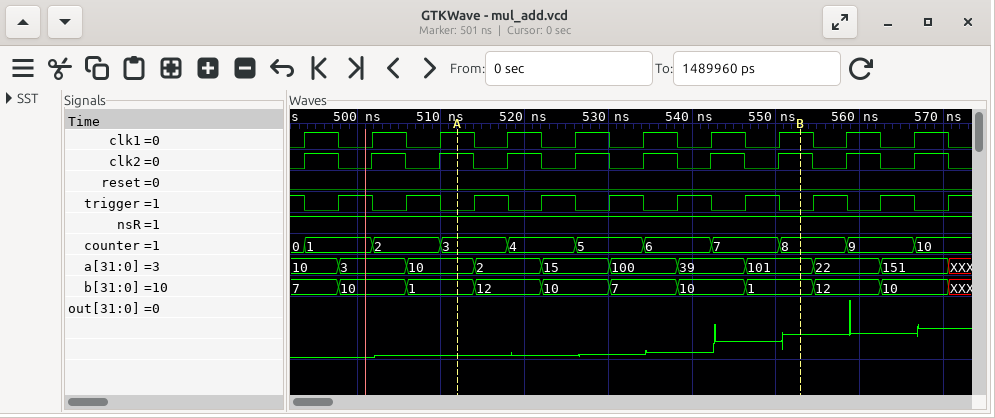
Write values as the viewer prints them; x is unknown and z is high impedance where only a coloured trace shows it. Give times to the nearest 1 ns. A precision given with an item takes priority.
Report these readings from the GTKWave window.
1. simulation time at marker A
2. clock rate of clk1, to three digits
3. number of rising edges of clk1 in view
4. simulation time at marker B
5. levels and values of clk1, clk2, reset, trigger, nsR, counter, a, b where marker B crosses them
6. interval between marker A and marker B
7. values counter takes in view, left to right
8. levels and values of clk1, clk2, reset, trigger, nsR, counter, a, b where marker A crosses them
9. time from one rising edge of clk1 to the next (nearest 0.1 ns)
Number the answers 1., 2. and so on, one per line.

1. 512 ns
2. 123 MHz
3. 10
4. 553 ns
5. clk1=1, clk2=1, reset=0, trigger=0, nsR=1, counter=8, a=101, b=1
6. 41 ns
7. 0, 1, 2, 3, 4, 5, 6, 7, 8, 9, 10
8. clk1=1, clk2=1, reset=0, trigger=0, nsR=1, counter=3, a=10, b=1
9. 8.1 ns
